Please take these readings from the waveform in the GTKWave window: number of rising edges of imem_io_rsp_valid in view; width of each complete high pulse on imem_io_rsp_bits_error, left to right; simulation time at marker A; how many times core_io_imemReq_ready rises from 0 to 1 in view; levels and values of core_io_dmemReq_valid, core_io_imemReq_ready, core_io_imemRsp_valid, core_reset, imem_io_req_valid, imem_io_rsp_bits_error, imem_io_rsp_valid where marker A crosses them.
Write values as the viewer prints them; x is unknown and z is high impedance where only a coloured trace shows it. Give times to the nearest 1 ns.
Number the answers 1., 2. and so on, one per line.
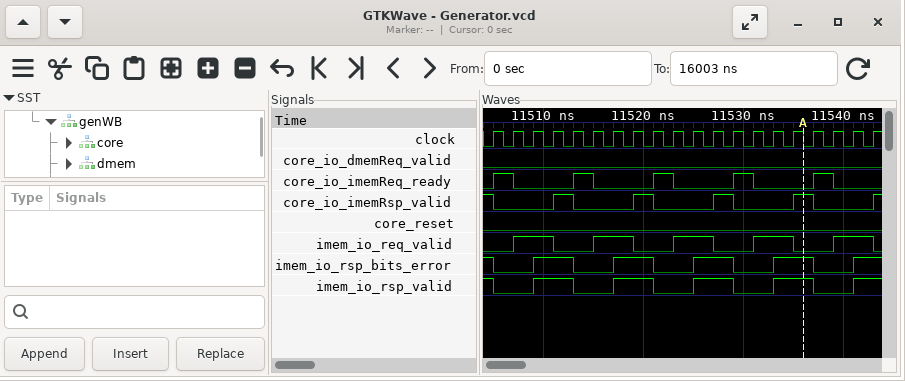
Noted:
1. 5
2. 4 ns, 4 ns, 4 ns, 4 ns
3. 11536 ns
4. 5
5. core_io_dmemReq_valid=0, core_io_imemReq_ready=0, core_io_imemRsp_valid=1, core_reset=0, imem_io_req_valid=0, imem_io_rsp_bits_error=1, imem_io_rsp_valid=1
